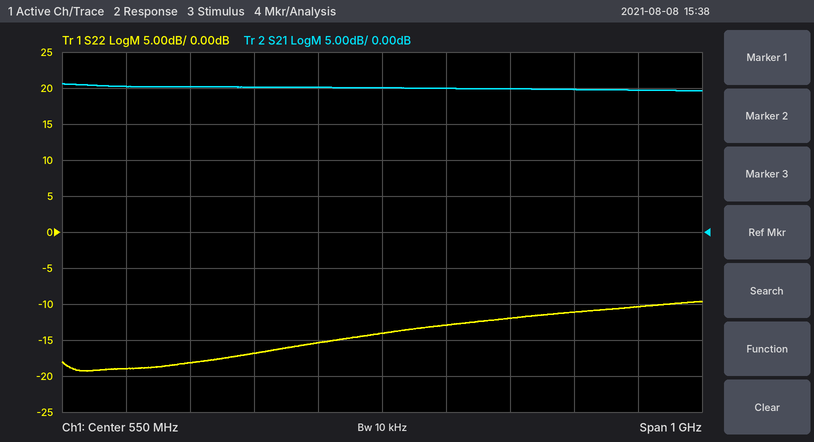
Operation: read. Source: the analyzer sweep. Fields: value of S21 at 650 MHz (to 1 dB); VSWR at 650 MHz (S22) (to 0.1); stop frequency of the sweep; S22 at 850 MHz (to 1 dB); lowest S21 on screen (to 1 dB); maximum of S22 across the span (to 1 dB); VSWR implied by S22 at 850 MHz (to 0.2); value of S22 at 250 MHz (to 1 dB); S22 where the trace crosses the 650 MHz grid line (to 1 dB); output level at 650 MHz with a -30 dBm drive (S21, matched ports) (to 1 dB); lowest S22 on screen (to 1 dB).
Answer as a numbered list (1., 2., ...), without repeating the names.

1. 20 dB
2. 1.6
3. 1.05 GHz
4. -11 dB
5. 20 dB
6. -10 dB
7. 1.8
8. -18 dB
9. -13 dB
10. -10 dBm
11. -19 dB
